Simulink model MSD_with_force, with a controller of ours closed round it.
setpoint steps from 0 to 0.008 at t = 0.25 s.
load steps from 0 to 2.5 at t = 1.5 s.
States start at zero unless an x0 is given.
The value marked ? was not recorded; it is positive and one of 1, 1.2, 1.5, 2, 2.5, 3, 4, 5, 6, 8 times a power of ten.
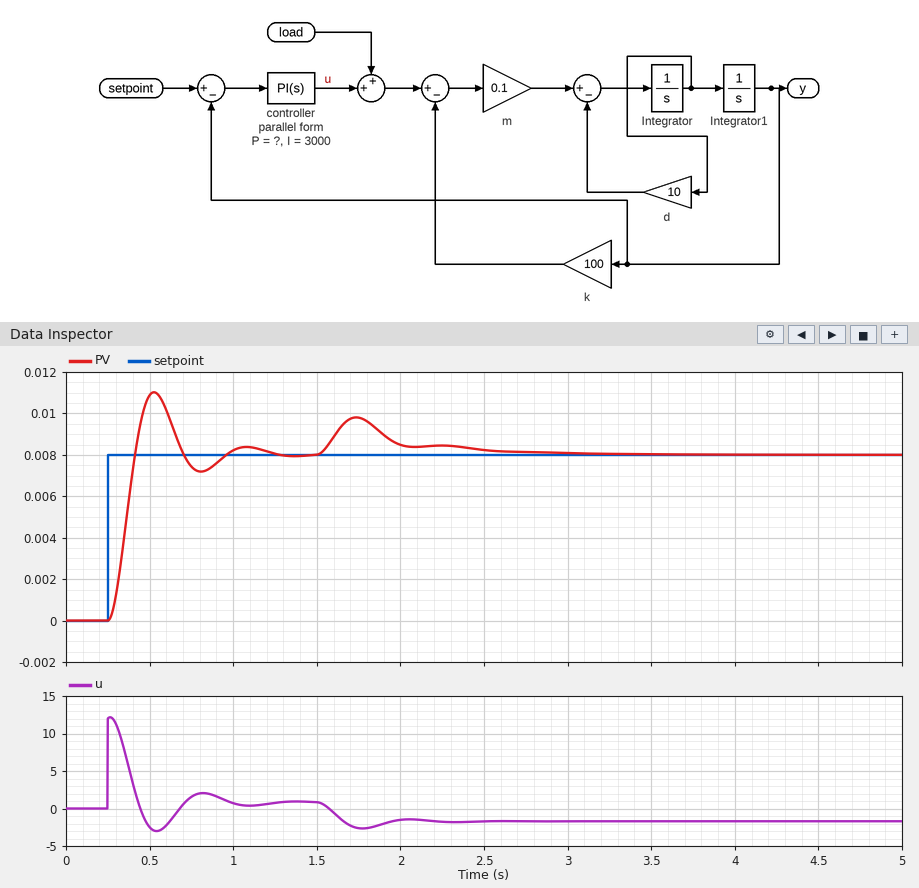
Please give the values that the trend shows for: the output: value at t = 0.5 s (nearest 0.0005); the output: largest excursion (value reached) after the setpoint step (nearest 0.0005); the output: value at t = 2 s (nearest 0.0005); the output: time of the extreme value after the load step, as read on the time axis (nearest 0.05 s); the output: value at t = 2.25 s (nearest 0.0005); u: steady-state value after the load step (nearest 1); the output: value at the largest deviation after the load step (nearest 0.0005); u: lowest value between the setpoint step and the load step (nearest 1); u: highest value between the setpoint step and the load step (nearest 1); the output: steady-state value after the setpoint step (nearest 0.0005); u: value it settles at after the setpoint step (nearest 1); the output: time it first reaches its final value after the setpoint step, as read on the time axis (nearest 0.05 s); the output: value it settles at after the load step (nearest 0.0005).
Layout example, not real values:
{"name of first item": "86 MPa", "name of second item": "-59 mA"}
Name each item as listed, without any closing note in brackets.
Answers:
{"the output: value at t = 0.5 s": "0.0110", "the output: largest excursion (value reached) after the setpoint step": "0.0110", "the output: value at t = 2 s": "0.0085", "the output: time of the extreme value after the load step, as read on the time axis": "1.75 s", "the output: value at t = 2.25 s": "0.0085", "u: steady-state value after the load step": "-2", "the output: value at the largest deviation after the load step": "0.0100", "u: lowest value between the setpoint step and the load step": "-3", "u: highest value between the setpoint step and the load step": "12", "the output: steady-state value after the setpoint step": "0.0080", "u: value it settles at after the setpoint step": "1", "the output: time it first reaches its final value after the setpoint step, as read on the time axis": "0.40 s", "the output: value it settles at after the load step": "0.0080"}
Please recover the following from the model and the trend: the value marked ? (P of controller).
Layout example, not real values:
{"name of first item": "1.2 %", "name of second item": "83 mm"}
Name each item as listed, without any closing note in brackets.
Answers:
{"the value marked ?": "1500"}
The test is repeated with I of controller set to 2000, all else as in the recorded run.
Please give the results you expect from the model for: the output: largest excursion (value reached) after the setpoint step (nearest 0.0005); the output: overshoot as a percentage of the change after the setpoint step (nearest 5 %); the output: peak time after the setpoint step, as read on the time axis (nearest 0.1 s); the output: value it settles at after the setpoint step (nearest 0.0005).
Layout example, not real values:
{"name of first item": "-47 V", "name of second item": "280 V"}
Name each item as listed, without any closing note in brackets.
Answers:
{"the output: largest excursion (value reached) after the setpoint step": "0.0105", "the output: overshoot as a percentage of the change after the setpoint step": "30 %", "the output: peak time after the setpoint step, as read on the time axis": "0.5 s", "the output: value it settles at after the setpoint step": "0.0080"}
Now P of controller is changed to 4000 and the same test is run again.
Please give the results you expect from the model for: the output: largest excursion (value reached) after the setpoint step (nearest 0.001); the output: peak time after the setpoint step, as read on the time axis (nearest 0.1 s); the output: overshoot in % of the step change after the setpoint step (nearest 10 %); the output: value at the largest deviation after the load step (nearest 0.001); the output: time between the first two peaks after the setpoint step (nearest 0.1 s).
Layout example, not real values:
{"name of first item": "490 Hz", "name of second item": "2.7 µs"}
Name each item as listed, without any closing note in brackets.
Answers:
{"the output: largest excursion (value reached) after the setpoint step": "0.012", "the output: peak time after the setpoint step, as read on the time axis": "0.4 s", "the output: overshoot in % of the step change after the setpoint step": "50 %", "the output: value at the largest deviation after the load step": "0.009", "the output: time between the first two peaks after the setpoint step": "0.3 s"}
